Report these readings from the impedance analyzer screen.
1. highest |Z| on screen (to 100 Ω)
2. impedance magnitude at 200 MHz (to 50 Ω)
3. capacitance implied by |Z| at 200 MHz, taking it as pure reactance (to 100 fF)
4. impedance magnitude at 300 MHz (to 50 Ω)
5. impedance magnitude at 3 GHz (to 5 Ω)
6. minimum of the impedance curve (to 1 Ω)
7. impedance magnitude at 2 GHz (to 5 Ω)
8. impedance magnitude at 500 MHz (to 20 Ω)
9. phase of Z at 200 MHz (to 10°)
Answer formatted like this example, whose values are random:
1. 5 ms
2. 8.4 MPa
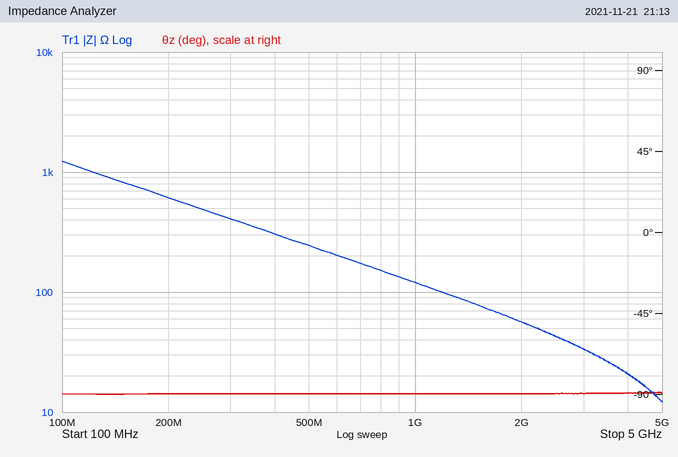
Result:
1. 1.2 kΩ
2. 600 Ω
3. 1.3 pF
4. 400 Ω
5. 35 Ω
6. 12 Ω
7. 55 Ω
8. 240 Ω
9. -90°
